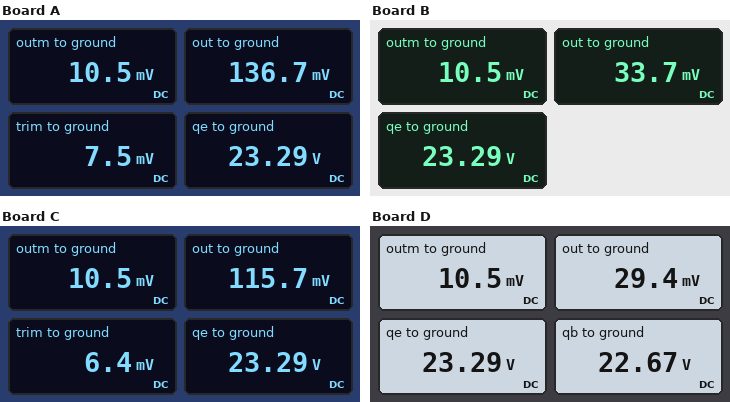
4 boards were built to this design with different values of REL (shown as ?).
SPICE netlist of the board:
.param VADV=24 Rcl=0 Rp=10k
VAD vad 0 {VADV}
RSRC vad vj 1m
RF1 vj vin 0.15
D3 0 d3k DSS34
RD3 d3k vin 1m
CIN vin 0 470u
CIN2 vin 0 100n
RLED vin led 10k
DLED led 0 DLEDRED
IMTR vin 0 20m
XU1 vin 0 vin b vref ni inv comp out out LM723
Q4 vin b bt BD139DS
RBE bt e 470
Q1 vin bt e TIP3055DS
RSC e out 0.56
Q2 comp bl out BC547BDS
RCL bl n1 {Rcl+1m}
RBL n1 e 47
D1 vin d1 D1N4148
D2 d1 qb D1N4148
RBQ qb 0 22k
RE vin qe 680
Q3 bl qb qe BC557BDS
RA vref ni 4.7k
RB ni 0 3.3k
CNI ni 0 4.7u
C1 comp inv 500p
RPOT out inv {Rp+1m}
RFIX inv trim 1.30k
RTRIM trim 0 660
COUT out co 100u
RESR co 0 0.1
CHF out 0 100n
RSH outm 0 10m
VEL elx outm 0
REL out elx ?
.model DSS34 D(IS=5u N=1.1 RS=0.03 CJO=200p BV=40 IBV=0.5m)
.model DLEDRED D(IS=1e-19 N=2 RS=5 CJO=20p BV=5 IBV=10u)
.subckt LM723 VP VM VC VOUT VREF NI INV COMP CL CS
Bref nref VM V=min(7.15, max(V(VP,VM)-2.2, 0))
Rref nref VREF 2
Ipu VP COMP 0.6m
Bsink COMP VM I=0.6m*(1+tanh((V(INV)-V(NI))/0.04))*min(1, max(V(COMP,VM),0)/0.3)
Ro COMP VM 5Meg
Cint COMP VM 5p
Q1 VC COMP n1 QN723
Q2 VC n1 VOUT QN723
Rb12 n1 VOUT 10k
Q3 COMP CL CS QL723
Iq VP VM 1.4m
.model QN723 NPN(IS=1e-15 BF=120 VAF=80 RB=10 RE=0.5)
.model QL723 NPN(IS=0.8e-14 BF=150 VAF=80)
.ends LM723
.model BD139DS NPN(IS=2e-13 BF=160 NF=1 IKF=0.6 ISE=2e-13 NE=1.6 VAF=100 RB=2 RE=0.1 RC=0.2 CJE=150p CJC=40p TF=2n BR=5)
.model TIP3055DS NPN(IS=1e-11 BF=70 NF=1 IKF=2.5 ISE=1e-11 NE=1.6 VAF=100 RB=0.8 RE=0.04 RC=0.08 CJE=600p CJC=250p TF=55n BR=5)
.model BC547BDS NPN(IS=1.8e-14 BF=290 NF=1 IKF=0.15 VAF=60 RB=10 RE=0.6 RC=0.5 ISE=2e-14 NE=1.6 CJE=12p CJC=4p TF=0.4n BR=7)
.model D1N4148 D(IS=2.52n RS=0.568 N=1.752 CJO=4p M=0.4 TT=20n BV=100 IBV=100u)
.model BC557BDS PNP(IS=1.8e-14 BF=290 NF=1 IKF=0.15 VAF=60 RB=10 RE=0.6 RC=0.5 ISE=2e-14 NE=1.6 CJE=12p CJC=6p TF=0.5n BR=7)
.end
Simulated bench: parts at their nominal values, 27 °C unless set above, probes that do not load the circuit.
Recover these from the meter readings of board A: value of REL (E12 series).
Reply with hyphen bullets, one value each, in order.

- 0.12 Ω
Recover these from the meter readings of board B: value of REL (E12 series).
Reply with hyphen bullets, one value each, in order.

- 0.022 Ω
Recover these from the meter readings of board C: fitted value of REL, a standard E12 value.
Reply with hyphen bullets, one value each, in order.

- 0.1 Ω
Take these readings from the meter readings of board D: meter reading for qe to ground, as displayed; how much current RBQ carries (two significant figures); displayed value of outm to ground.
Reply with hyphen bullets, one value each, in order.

- 23.29 V
- 1.0 mA
- 10.5 mV
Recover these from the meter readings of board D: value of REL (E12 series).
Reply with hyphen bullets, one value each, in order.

- 0.018 Ω
